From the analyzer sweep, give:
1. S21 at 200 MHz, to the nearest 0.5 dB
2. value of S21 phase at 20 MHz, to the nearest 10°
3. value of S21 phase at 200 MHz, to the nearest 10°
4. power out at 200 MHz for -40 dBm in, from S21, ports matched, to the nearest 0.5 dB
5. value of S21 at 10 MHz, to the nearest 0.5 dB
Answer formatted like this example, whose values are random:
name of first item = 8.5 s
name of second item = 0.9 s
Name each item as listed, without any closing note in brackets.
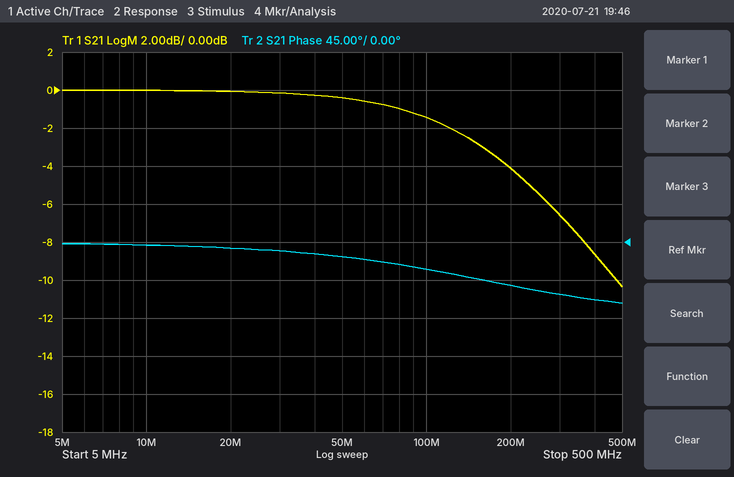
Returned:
S21 at 200 MHz, to the nearest 0.5 dB = -4.0 dB
value of S21 phase at 20 MHz, to the nearest 10° = -10°
value of S21 phase at 200 MHz, to the nearest 10° = -50°
power out at 200 MHz for -40 dBm in, from S21, ports matched, to the nearest 0.5 dB = -44.0 dBm
value of S21 at 10 MHz, to the nearest 0.5 dB = 0.0 dB
